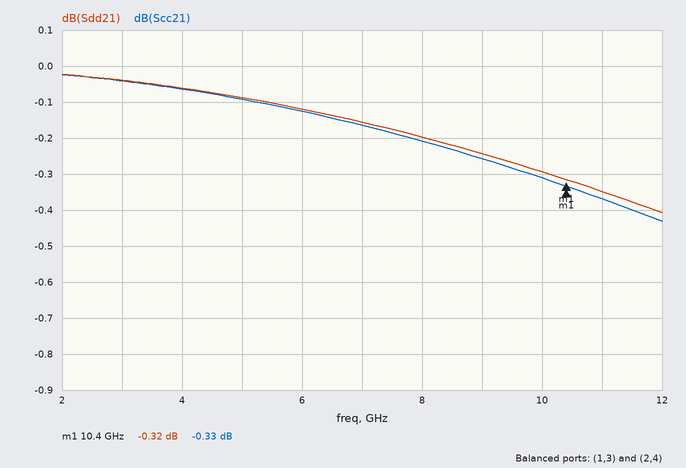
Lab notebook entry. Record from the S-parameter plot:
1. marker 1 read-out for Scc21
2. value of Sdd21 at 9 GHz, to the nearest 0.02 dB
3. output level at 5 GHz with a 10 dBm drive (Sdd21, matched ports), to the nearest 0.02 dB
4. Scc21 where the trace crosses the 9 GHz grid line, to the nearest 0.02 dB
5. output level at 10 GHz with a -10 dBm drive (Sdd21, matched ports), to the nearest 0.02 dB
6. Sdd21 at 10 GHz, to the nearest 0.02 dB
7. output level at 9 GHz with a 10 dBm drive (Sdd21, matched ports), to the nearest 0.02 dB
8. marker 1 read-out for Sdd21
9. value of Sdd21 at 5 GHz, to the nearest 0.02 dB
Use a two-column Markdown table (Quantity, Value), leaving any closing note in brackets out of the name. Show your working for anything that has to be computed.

| Quantity | Value |
|---|---|
| marker 1 read-out for Scc21 | -0.33 dB |
| value of Sdd21 at 9 GHz, to the nearest 0.02 dB | -0.24 dB |
| output level at 5 GHz with a 10 dBm drive (Sdd21, matched ports), to the nearest 0.02 dB | 10 dBm + (-0.08 dB) = 9.92 dBm |
| Scc21 where the trace crosses the 9 GHz grid line, to the nearest 0.02 dB | -0.26 dB |
| output level at 10 GHz with a -10 dBm drive (Sdd21, matched ports), to the nearest 0.02 dB | -10 dBm + (-0.30 dB) = -10.30 dBm |
| Sdd21 at 10 GHz, to the nearest 0.02 dB | -0.30 dB |
| output level at 9 GHz with a 10 dBm drive (Sdd21, matched ports), to the nearest 0.02 dB | 10 dBm + (-0.24 dB) = 9.76 dBm |
| marker 1 read-out for Sdd21 | -0.32 dB |
| value of Sdd21 at 5 GHz, to the nearest 0.02 dB | -0.08 dB |
